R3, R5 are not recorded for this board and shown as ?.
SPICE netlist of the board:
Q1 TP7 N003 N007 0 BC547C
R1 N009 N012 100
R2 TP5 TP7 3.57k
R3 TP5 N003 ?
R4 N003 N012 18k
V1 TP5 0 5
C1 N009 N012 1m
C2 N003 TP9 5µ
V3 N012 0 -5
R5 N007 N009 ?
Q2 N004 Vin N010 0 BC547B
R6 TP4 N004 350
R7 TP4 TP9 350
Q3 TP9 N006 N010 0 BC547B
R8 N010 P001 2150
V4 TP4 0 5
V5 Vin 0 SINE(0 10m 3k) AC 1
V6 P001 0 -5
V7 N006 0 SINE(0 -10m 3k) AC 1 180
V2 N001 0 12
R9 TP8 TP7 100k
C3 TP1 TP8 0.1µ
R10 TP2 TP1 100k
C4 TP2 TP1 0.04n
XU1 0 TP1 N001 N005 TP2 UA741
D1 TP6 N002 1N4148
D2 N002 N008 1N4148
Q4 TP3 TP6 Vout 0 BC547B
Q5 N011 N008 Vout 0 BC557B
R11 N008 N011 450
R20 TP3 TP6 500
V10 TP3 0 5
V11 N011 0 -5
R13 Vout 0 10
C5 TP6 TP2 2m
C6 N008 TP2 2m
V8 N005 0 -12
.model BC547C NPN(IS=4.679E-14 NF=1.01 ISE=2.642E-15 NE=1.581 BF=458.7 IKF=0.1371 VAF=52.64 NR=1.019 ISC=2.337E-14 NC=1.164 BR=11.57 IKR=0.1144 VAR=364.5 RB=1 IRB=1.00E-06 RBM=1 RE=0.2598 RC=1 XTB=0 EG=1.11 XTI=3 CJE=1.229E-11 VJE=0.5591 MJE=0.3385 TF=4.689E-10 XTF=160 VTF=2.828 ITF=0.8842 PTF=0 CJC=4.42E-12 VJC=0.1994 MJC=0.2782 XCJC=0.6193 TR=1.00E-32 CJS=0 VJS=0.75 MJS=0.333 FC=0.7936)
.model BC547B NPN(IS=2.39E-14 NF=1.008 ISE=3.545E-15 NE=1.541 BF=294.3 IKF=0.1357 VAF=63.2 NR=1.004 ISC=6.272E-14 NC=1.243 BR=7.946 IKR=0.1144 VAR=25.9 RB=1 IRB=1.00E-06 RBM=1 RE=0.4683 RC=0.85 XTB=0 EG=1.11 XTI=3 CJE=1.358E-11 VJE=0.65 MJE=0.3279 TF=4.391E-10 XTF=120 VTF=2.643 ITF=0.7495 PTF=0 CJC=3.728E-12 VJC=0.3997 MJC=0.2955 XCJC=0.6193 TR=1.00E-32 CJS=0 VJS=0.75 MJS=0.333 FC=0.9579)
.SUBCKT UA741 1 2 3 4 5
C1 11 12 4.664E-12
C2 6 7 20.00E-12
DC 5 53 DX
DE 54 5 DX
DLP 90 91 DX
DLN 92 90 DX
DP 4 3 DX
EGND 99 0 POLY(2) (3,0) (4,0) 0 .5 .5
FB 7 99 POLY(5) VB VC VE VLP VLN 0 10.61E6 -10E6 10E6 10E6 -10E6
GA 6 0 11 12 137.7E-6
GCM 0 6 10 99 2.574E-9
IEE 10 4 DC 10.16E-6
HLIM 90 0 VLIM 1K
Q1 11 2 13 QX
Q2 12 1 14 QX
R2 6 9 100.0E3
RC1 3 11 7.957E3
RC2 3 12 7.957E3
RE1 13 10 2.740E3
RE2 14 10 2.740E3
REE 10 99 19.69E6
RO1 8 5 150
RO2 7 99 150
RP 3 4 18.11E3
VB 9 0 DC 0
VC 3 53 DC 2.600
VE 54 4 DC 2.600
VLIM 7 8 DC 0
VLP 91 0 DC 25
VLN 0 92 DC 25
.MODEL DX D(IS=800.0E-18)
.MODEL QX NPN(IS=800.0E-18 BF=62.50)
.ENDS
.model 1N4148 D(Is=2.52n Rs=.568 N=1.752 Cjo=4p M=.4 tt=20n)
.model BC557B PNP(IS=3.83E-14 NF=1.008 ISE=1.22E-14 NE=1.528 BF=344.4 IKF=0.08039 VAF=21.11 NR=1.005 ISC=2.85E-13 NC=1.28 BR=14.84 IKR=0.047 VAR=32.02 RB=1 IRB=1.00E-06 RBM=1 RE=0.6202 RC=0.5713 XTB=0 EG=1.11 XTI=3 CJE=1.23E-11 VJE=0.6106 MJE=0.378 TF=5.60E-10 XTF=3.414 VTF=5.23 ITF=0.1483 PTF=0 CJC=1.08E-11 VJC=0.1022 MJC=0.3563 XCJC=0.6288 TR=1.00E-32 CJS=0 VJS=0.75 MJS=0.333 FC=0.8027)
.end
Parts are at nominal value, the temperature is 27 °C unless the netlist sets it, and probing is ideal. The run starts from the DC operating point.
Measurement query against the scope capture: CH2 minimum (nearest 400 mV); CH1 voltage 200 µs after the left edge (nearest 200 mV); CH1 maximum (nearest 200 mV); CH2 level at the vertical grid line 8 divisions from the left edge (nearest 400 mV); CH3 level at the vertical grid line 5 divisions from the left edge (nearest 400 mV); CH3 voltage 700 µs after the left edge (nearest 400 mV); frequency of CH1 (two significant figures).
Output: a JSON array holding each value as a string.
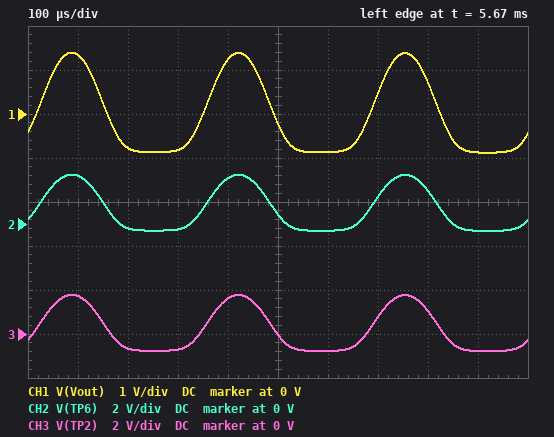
["-400 mV", "-800 mV", "1.4 V", "1.6 V", "0 V", "800 mV", "3.0 kHz"]
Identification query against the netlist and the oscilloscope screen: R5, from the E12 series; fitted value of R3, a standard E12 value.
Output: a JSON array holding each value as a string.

["150 Ω", "270 kΩ"]
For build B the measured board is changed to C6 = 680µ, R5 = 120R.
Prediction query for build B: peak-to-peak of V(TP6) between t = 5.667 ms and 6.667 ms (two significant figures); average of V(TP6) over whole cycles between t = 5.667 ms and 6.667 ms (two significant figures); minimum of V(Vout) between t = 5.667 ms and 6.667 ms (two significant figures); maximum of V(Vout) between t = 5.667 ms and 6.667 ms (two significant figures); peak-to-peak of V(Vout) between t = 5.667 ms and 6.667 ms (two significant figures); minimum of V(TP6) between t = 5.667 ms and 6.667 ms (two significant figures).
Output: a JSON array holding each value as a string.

["3.0 V", "710 mV", "-970 mV", "1.7 V", "2.7 V", "-410 mV"]
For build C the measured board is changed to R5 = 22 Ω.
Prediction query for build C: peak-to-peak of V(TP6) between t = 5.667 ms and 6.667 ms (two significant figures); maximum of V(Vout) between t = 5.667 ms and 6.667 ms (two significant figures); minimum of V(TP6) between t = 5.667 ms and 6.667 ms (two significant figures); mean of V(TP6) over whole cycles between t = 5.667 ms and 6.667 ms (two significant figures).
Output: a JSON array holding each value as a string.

["6.4 V", "4.1 V", "-1.3 V", "1.2 V"]
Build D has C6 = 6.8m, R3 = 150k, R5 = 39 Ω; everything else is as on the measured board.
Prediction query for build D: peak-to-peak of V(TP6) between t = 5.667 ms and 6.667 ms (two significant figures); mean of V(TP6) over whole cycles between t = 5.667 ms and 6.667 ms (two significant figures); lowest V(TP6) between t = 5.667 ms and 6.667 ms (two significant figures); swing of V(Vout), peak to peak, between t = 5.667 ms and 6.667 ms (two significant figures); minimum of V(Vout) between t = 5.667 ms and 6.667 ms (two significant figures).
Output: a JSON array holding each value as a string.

["6.3 V", "-860 mV", "-3.8 V", "5.7 V", "-4.1 V"]
